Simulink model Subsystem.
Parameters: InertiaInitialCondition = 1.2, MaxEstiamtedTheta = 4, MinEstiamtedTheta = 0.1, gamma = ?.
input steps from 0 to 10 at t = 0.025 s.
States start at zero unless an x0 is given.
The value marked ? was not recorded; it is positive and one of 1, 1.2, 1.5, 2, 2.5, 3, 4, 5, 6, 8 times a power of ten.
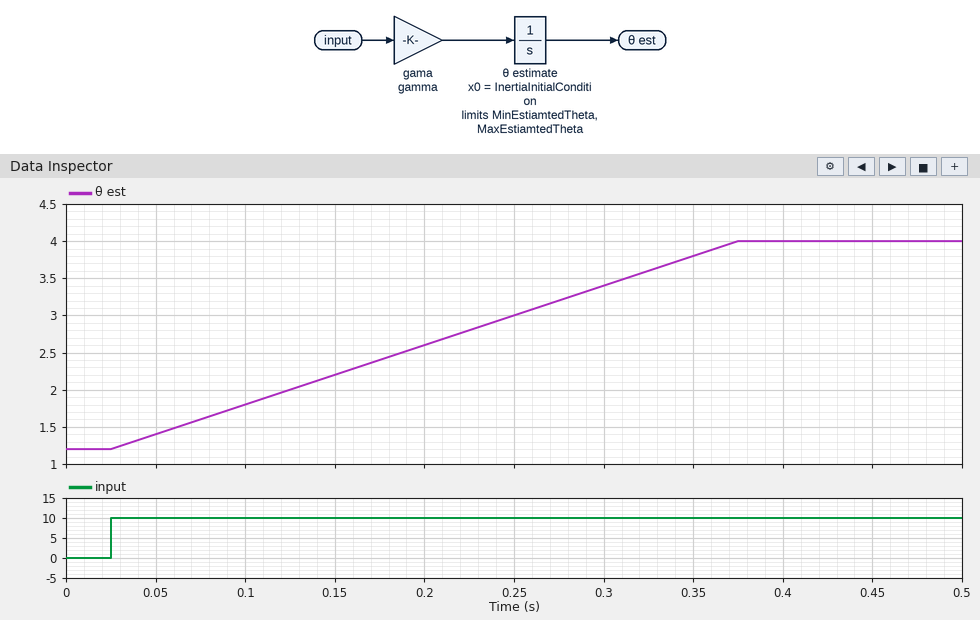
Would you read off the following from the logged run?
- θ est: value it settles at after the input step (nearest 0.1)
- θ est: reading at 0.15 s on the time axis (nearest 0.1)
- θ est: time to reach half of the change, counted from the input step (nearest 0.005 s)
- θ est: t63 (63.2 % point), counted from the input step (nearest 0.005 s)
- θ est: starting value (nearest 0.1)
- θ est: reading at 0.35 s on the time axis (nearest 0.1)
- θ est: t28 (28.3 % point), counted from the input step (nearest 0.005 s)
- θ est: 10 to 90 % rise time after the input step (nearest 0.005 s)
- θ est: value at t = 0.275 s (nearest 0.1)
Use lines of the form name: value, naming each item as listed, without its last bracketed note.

θ est: value it settles at after the input step: 4.0
θ est: reading at 0.15 s on the time axis: 2.2
θ est: time to reach half of the change, counted from the input step: 0.175 s
θ est: t63 (63.2 % point), counted from the input step: 0.220 s
θ est: starting value: 1.2
θ est: reading at 0.35 s on the time axis: 3.8
θ est: t28 (28.3 % point), counted from the input step: 0.100 s
θ est: 10 to 90 % rise time after the input step: 0.280 s
θ est: value at t = 0.275 s: 3.2
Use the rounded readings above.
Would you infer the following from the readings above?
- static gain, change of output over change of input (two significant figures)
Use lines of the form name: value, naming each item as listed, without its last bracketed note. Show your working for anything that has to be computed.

static gain, change of output over change of input: (4 - 1.2) / (10 - 0) = 0.28
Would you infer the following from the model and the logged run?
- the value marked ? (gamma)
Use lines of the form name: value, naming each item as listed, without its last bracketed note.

the value marked ?: 0.8
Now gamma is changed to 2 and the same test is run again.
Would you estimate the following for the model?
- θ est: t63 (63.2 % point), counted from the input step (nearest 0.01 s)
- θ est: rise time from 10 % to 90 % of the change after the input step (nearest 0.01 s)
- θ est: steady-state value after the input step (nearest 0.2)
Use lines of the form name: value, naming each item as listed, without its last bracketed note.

θ est: t63 (63.2 % point), counted from the input step: 0.09 s
θ est: rise time from 10 % to 90 % of the change after the input step: 0.11 s
θ est: steady-state value after the input step: 4.0
